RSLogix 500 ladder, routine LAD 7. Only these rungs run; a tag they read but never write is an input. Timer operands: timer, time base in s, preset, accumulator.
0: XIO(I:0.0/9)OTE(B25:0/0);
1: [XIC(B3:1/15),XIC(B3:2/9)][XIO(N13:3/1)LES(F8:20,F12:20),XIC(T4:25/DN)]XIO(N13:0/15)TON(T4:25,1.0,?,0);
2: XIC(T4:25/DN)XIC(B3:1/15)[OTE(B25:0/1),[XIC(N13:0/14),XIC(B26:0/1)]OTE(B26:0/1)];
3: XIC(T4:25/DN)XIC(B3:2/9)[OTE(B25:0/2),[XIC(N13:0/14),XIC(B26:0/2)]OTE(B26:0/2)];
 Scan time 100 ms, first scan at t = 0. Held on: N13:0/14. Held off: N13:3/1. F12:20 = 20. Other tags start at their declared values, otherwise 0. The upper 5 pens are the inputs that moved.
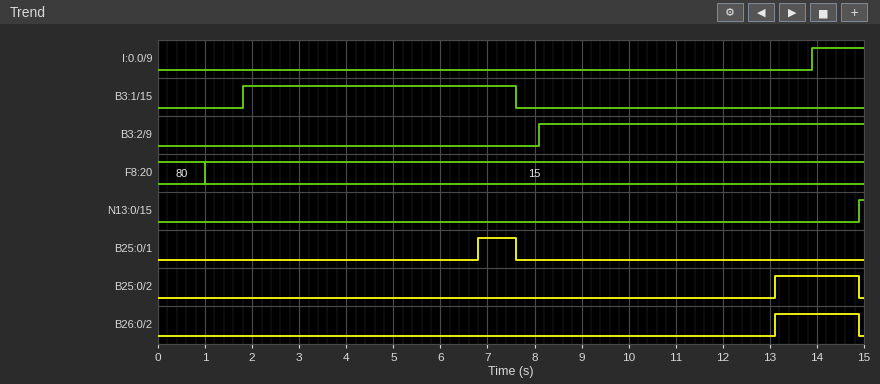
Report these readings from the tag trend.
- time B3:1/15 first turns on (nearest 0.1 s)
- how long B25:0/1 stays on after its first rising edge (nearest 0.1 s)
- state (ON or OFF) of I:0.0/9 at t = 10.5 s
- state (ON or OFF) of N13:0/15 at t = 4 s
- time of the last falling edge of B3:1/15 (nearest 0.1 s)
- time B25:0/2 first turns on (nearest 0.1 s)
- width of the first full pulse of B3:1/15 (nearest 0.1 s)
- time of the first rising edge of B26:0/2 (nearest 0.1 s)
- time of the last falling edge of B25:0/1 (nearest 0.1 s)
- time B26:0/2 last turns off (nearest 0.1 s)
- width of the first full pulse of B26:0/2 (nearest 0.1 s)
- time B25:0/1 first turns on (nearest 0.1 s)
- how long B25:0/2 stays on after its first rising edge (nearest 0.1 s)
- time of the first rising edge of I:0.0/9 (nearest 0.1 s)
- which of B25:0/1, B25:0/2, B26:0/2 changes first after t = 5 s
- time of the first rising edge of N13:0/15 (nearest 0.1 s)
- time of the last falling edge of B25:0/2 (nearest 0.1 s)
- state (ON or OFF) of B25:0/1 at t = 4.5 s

1.8 s
0.8 s
OFF
OFF
7.6 s
13.1 s
5.8 s
13.1 s
7.6 s
14.9 s
1.8 s
6.8 s
1.8 s
13.9 s
B25:0/1
14.9 s
14.9 s
OFF
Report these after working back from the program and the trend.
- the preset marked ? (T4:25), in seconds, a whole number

5 s
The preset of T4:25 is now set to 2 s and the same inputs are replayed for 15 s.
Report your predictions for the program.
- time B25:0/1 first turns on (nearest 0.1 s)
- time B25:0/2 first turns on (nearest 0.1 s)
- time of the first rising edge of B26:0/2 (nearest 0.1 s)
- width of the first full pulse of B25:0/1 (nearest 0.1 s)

3.8 s
10.1 s
10.1 s
3.8 s
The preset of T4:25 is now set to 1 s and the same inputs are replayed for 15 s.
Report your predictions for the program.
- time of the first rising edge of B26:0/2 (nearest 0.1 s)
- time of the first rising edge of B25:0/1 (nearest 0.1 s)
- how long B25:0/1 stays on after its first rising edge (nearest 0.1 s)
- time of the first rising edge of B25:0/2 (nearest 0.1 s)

9.1 s
2.8 s
4.8 s
9.1 s
